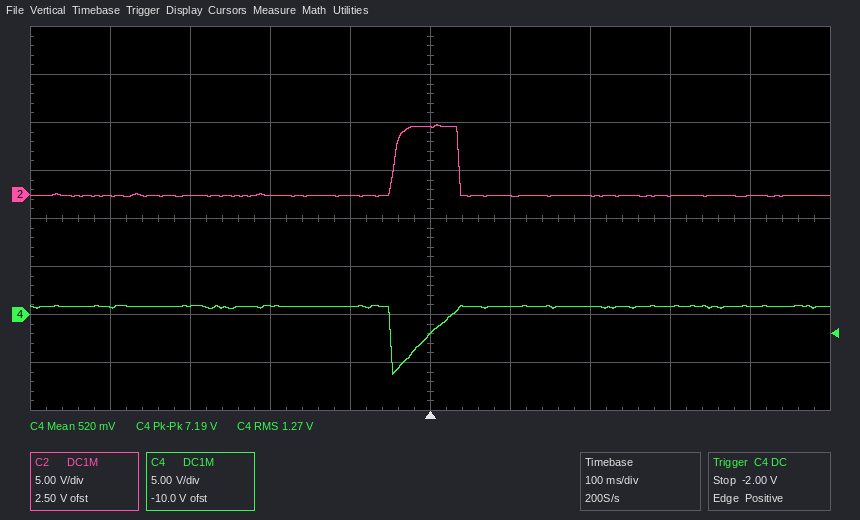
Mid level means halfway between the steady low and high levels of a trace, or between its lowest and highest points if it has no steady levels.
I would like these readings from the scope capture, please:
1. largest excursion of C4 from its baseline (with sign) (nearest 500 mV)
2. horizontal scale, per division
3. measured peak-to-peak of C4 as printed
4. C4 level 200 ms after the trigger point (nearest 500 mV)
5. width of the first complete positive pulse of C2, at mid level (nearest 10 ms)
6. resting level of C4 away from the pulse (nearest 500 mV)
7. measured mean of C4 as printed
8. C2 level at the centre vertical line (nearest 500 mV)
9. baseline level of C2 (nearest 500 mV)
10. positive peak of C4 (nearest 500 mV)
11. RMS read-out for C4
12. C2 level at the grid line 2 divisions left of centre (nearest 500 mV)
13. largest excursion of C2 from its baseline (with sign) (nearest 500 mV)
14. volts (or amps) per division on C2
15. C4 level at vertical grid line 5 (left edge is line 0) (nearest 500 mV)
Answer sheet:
-7.0 V
100 ms
7.19 V
1.0 V
80 ms
1.0 V
520 mV
7.0 V
0.0 V
1.0 V
1.27 V
0.0 V
+7.5 V
5 V
-2.0 V
